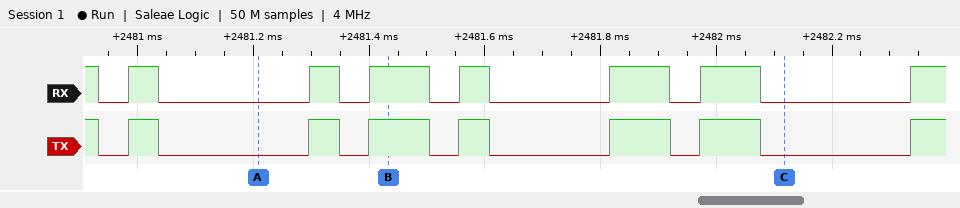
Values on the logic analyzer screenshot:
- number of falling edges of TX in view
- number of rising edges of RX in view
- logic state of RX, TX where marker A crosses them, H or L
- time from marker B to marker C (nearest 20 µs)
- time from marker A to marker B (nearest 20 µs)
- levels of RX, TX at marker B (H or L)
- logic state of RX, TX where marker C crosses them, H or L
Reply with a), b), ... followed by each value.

a) 7
b) 7
c) RX=L, TX=L
d) 680 µs
e) 220 µs
f) RX=H, TX=H
g) RX=L, TX=L
